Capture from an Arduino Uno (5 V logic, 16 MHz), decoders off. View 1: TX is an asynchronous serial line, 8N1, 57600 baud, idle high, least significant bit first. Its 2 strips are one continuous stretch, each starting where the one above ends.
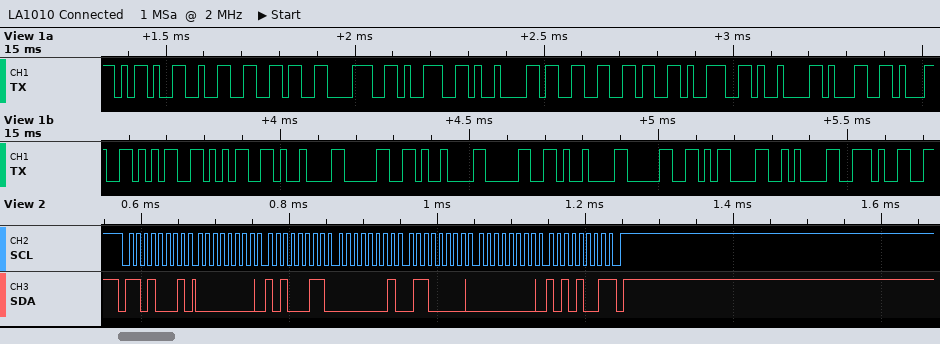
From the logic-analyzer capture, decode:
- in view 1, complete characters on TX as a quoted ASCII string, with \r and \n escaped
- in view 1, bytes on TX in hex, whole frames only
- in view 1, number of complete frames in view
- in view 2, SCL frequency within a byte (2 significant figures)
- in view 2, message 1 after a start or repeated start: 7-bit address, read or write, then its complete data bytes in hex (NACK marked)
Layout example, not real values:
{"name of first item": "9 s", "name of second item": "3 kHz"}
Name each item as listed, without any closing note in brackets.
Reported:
{"in view 1, complete characters on TX as a quoted ASCII string, with \\r and \\n escaped": "\"-2689\\t369\\t1155\\t0\\t0\\t0\\r\\n.\"", "in view 1, bytes on TX in hex, whole frames only": "2D 32 36 38 39 09 33 36 39 09 31 31 35 35 09 30 09 30 09 30 0D 0A 2E", "in view 1, number of complete frames in view": "23", "in view 2, SCL frequency within a byte": "100 kHz", "in view 2, message 1 after a start or repeated start: 7-bit address, read or write, then its complete data bytes in hex": "0x68 read: 00 A3 01 60 00 A9 NACK"}
